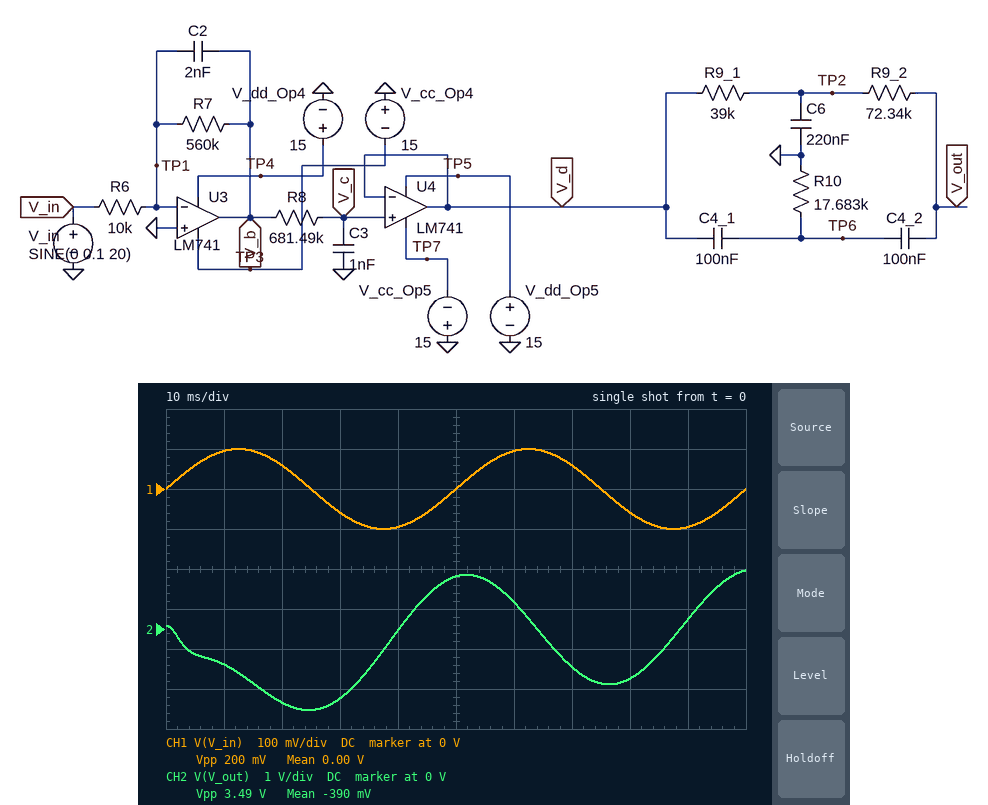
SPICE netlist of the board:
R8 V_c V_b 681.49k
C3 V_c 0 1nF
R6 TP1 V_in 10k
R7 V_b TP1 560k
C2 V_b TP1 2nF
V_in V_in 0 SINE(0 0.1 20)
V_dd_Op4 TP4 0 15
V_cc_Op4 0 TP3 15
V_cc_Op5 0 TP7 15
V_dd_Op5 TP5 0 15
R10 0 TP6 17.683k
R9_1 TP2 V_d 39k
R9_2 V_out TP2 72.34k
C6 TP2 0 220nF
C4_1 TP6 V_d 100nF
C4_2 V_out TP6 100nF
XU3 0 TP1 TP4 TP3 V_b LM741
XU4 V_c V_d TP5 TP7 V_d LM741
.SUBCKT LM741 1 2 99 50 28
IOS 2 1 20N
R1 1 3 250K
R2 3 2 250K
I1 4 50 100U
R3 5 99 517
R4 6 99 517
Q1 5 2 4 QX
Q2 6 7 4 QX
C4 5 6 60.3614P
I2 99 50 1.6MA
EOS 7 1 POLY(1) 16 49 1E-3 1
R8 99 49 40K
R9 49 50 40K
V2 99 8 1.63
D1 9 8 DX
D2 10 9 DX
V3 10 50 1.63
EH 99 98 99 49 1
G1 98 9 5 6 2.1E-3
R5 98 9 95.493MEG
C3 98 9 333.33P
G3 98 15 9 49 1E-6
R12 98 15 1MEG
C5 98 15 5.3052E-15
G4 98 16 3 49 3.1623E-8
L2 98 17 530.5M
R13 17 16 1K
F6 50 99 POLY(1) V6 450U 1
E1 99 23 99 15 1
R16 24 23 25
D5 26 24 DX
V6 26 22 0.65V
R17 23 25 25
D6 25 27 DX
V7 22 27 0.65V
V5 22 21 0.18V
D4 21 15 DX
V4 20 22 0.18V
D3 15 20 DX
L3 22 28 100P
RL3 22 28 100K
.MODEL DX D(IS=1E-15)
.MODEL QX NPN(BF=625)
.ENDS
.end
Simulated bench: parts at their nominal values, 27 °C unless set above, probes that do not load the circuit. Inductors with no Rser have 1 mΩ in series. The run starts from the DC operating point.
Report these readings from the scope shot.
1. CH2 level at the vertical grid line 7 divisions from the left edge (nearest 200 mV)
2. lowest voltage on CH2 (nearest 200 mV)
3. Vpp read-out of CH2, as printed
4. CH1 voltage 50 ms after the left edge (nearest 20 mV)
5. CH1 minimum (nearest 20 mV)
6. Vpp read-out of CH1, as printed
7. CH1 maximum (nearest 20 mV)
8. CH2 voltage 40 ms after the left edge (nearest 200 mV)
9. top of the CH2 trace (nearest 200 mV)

-1.0 V
-2.0 V
3.49 V
0 V
-100 mV
200 mV
100 mV
0 V
1.4 V
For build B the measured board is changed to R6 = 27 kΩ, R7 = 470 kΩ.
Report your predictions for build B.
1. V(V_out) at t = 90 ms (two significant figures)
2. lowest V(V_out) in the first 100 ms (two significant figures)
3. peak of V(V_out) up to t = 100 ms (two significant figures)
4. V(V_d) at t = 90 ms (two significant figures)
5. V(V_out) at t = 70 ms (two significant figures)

90 mV
-630 mV
460 mV
1.7 V
-300 mV
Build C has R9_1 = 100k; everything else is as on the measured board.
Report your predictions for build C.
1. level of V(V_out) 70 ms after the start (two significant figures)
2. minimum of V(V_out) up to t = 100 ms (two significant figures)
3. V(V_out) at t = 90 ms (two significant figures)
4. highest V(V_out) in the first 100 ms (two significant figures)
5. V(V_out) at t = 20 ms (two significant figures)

-80 mV
-1.0 V
-370 mV
310 mV
-700 mV
